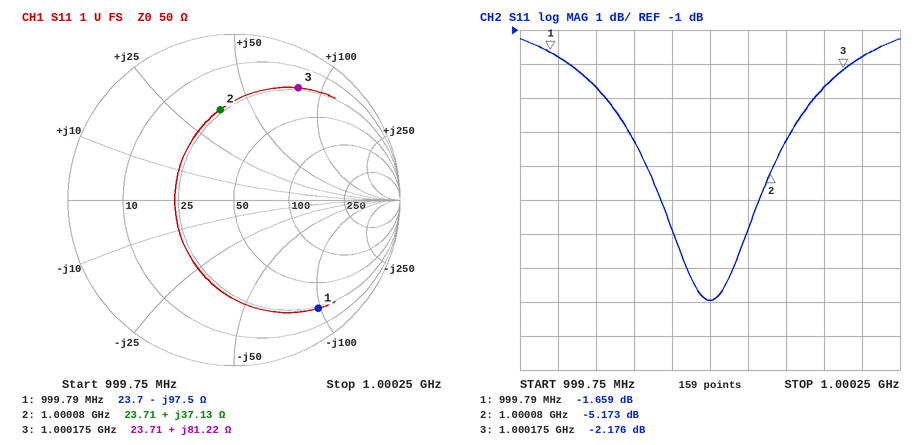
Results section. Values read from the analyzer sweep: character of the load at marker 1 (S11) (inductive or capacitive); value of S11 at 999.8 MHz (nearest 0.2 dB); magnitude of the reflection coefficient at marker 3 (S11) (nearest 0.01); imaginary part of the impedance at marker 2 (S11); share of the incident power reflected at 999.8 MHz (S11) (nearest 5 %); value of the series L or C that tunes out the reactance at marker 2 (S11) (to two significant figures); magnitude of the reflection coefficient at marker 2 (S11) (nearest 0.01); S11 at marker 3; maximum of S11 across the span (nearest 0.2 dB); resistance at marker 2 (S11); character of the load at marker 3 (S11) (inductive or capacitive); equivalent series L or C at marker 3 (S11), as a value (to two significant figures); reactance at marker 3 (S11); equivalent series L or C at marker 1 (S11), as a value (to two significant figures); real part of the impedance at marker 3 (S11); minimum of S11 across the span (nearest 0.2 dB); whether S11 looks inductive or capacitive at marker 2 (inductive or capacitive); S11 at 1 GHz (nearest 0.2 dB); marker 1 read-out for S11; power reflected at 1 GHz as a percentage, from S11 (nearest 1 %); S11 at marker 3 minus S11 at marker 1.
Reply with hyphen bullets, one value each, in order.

- capacitive
- -1.8 dB
- 0.78
- +37.13 Ω
- 65 %
- 4.3 pF
- 0.55
- -2.176 dB
- -1.2 dB
- 23.71 Ω
- inductive
- 13 nH
- +81.22 Ω
- 1.6 pF
- 23.71 Ω
- -9.0 dB
- inductive
- -9.0 dB
- -1.659 dB
- 13 %
- -0.517 dB
